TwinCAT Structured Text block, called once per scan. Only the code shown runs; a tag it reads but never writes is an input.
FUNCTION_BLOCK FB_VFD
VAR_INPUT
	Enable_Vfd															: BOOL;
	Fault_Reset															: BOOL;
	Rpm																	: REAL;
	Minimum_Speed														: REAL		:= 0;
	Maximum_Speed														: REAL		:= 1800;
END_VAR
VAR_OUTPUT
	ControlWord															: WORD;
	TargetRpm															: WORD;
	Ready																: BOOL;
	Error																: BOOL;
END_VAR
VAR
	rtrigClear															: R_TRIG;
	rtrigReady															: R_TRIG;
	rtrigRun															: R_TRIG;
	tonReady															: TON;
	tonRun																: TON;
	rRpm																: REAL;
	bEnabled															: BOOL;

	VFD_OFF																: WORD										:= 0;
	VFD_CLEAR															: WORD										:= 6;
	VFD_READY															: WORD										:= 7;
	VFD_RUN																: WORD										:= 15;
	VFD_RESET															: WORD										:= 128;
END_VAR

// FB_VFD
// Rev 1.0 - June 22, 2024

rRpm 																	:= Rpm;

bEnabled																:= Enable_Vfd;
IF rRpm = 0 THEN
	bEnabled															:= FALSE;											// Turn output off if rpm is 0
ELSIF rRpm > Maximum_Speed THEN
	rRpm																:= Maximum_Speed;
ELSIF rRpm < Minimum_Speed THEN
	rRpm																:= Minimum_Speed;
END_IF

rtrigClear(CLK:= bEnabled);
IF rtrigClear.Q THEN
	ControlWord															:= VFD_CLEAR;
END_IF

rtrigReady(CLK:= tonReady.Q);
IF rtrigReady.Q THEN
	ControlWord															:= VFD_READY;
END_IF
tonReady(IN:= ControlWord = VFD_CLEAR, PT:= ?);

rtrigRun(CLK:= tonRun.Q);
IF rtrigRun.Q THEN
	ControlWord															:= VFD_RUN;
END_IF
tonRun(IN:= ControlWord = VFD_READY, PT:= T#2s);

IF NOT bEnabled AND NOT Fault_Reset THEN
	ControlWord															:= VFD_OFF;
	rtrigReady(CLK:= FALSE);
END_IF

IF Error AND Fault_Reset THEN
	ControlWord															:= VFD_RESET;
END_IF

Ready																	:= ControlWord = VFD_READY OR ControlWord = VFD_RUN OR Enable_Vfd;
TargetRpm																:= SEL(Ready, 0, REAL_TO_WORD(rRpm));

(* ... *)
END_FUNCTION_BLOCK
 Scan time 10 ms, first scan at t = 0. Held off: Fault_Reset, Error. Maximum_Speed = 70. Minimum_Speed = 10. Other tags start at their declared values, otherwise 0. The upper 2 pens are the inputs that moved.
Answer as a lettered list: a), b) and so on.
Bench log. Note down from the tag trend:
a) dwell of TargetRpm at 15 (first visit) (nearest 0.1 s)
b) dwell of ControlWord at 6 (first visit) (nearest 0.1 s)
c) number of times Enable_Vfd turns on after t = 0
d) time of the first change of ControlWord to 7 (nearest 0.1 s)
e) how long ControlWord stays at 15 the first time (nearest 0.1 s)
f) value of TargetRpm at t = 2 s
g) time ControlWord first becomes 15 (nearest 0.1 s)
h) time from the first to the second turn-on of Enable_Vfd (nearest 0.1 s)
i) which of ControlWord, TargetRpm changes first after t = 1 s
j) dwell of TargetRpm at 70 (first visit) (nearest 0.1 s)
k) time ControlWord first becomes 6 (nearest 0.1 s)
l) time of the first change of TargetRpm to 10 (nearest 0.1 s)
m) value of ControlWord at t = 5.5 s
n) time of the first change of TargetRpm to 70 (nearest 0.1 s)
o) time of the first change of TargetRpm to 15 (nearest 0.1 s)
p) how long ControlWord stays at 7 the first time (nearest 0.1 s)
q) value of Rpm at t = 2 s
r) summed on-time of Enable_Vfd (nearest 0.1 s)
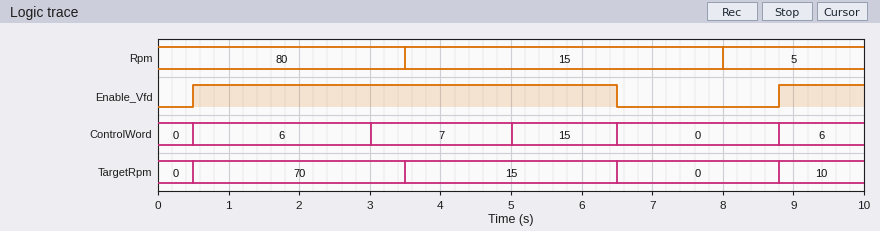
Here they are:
a) 3.0 s
b) 2.5 s
c) 2
d) 3.0 s
e) 1.5 s
f) 70
g) 5.0 s
h) 8.3 s
i) ControlWord
j) 3.0 s
k) 0.5 s
l) 8.8 s
m) 15
n) 0.5 s
o) 3.5 s
p) 2.0 s
q) 80
r) 7.2 s
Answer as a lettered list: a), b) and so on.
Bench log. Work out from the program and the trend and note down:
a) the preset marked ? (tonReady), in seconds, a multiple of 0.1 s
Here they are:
a) 2.5 s
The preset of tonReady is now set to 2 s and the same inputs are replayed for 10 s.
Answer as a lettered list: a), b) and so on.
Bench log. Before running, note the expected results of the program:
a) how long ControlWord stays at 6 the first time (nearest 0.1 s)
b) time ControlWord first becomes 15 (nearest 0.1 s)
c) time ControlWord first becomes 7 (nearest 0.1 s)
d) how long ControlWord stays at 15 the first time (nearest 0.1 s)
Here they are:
a) 2.0 s
b) 4.5 s
c) 2.5 s
d) 2.0 s
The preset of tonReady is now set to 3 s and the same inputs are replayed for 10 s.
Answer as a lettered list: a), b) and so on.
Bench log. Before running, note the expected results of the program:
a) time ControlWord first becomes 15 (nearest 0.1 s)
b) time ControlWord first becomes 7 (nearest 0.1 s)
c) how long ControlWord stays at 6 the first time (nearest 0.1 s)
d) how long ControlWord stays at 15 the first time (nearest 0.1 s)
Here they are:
a) 5.5 s
b) 3.5 s
c) 3.0 s
d) 1.0 s
